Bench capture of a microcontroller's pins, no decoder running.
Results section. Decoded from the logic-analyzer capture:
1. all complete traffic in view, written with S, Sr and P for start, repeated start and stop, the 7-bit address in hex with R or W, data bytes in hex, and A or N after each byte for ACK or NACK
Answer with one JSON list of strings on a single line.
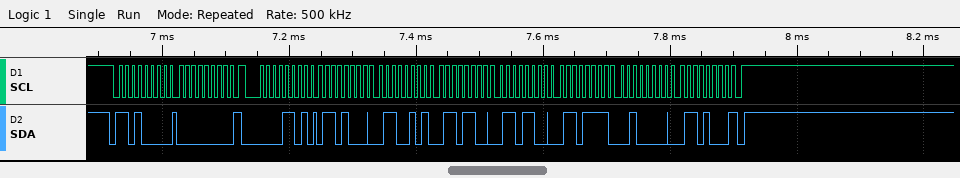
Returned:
["S 68W A 00 A Sr 06R A 68 A 65 A 6C A 6C A 6F A 20 A 68 N P"]
